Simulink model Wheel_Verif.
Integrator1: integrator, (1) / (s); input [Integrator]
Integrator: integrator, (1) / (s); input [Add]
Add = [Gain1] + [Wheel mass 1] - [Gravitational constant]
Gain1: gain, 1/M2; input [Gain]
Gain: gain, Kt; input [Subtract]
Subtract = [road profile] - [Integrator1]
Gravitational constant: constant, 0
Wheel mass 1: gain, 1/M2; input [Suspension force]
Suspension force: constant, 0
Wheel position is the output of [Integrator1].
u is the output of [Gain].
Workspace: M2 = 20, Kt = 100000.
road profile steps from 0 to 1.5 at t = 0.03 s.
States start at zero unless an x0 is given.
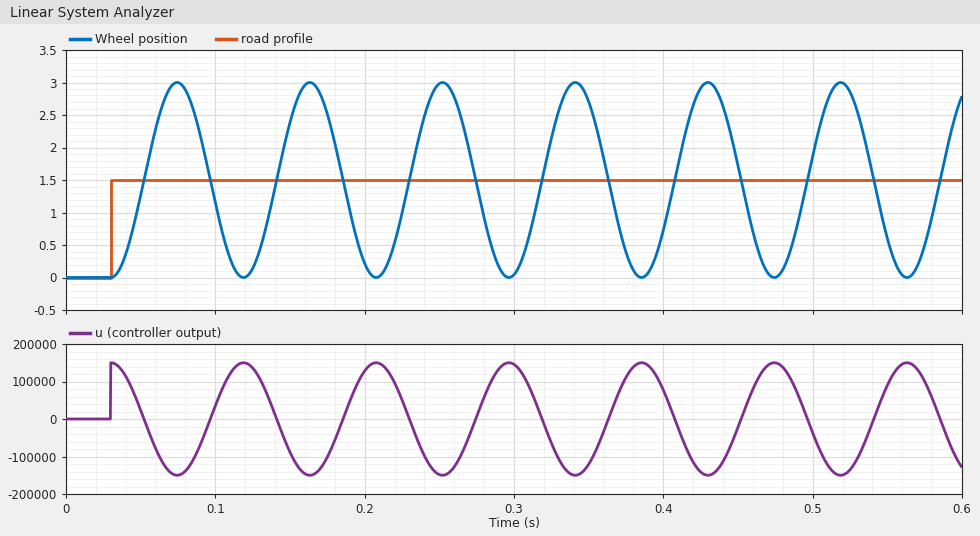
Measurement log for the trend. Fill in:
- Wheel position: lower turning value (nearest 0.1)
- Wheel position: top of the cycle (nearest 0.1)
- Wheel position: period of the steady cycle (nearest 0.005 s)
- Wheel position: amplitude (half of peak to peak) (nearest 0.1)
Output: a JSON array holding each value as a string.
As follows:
["0.0", "3.0", "0.090 s", "1.5"]
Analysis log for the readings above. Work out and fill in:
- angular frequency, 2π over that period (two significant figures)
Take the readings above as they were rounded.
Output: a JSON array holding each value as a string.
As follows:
["70 rad/s"]
